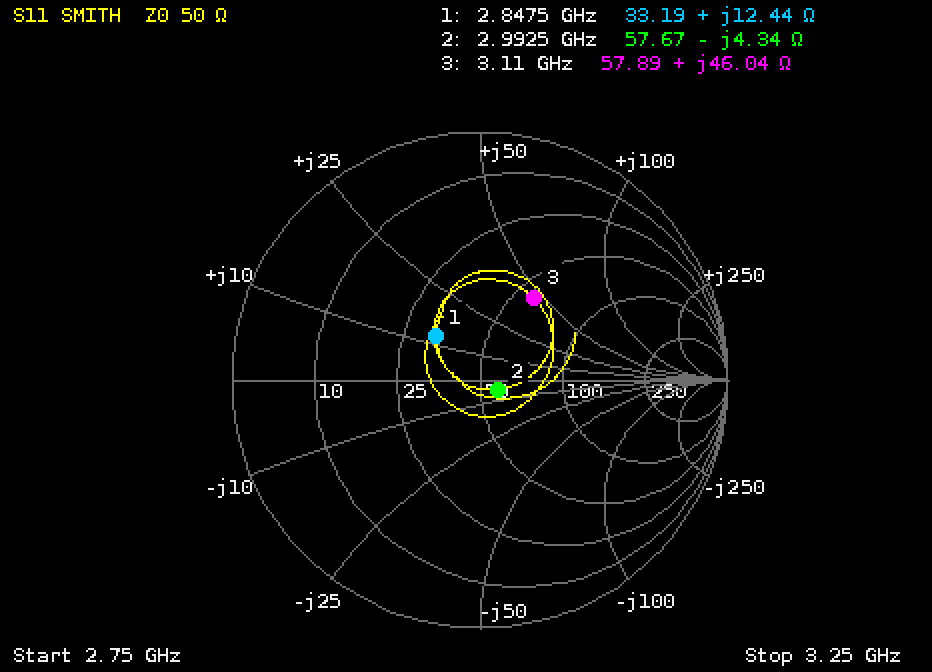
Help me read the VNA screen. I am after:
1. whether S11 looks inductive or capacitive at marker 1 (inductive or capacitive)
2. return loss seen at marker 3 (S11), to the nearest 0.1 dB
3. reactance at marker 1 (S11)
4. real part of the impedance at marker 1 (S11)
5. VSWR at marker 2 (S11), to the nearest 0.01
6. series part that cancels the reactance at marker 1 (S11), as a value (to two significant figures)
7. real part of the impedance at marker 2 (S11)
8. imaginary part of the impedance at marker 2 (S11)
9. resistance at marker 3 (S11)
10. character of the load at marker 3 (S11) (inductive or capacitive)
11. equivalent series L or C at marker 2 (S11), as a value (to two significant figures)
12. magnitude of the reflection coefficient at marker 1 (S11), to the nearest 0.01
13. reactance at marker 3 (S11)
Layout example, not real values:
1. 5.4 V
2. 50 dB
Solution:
1. inductive
2. 8.0 dB
3. +12.44 Ω
4. 33.19 Ω
5. 1.18
6. 4.5 pF
7. 57.67 Ω
8. -4.34 Ω
9. 57.89 Ω
10. inductive
11. 12 pF
12. 0.25
13. +46.04 Ω
